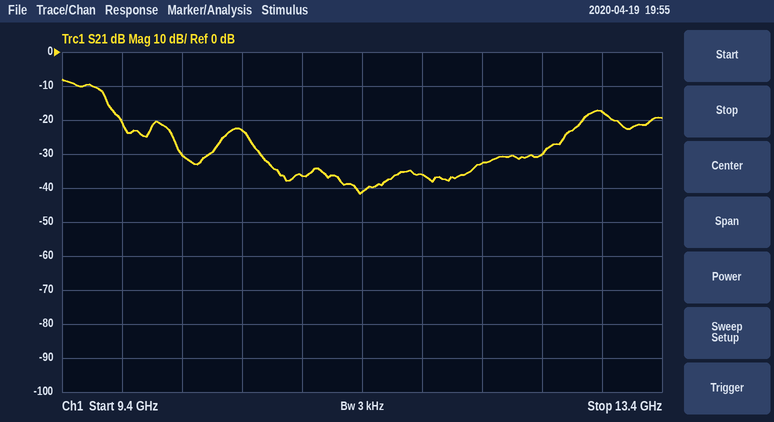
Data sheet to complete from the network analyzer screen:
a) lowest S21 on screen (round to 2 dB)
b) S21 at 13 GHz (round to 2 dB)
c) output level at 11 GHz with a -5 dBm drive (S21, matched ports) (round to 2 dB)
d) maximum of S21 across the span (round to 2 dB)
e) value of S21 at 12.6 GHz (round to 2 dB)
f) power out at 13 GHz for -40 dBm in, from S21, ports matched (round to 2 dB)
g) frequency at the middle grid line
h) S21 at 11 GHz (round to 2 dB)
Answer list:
-42 dB
-18 dB
-42 dBm
-8 dB
-30 dB
-58 dBm
11.4 GHz
-36 dB
